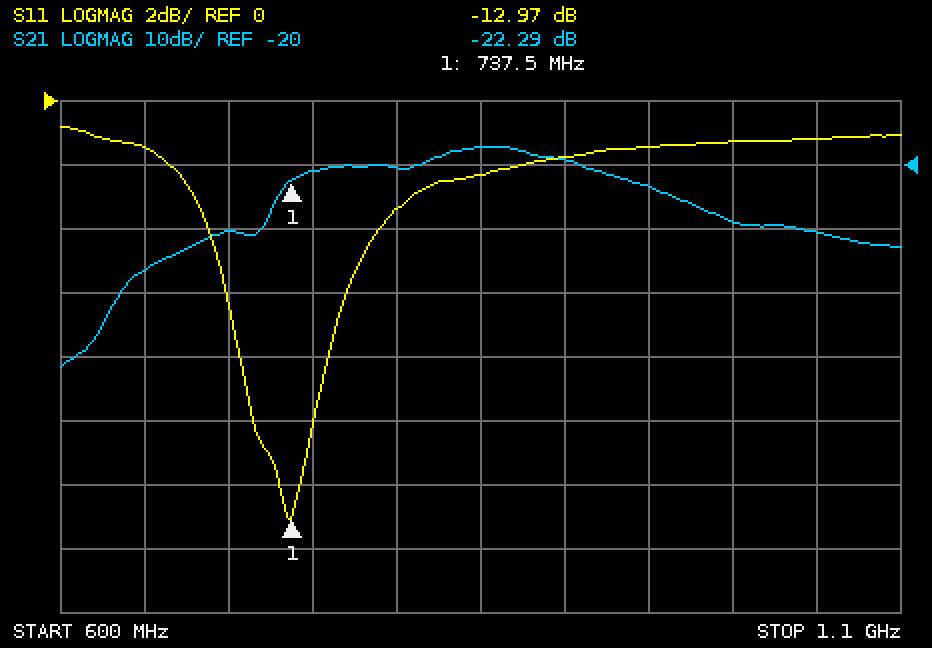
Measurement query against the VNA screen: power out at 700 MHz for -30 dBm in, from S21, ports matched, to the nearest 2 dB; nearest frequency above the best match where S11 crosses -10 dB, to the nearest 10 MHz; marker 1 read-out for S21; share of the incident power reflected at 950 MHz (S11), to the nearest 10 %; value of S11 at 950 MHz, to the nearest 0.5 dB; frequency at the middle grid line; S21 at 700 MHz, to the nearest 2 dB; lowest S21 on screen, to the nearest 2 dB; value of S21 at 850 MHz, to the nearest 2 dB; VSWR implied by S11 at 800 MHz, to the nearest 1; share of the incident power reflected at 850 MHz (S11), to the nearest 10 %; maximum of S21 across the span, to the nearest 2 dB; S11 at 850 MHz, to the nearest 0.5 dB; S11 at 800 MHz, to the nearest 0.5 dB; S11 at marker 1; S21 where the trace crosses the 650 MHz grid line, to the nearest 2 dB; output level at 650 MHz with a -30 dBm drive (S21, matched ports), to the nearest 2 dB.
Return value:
-60 dBm
750 MHz
-22.29 dB
70 %
-1.5 dB
850 MHz
-30 dB
-52 dB
-18 dB
5
60 %
-18 dB
-2.5 dB
-3.5 dB
-12.97 dB
-36 dB
-66 dBm
